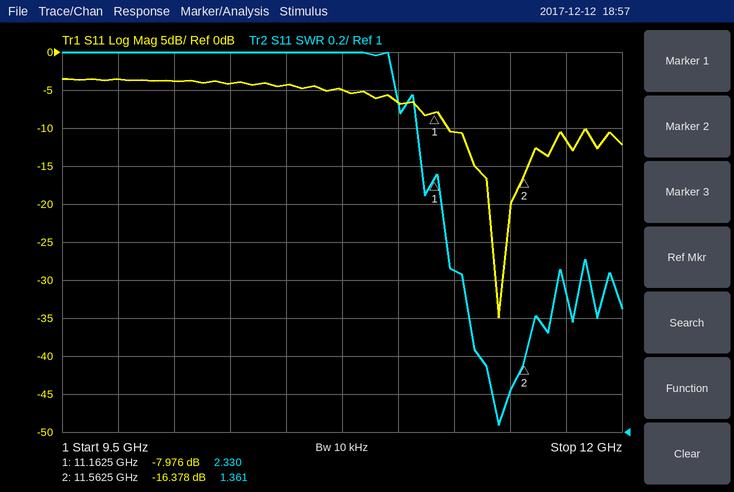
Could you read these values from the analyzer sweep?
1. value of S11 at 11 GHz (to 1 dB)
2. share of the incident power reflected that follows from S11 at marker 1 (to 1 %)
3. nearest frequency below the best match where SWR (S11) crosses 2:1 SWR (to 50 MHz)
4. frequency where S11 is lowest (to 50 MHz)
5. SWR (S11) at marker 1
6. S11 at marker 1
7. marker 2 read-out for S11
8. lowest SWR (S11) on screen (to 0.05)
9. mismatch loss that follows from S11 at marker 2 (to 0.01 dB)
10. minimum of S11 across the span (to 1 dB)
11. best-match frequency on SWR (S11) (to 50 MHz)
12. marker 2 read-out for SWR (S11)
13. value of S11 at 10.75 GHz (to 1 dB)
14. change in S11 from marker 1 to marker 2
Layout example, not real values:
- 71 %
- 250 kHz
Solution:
- -7 dB
- 16 %
- 11.20 GHz
- 11.45 GHz
- 2.330
- -7.976 dB
- -16.378 dB
- 1.05
- 0.10 dB
- -35 dB
- 11.45 GHz
- 1.361
- -5 dB
- -8.402 dB
